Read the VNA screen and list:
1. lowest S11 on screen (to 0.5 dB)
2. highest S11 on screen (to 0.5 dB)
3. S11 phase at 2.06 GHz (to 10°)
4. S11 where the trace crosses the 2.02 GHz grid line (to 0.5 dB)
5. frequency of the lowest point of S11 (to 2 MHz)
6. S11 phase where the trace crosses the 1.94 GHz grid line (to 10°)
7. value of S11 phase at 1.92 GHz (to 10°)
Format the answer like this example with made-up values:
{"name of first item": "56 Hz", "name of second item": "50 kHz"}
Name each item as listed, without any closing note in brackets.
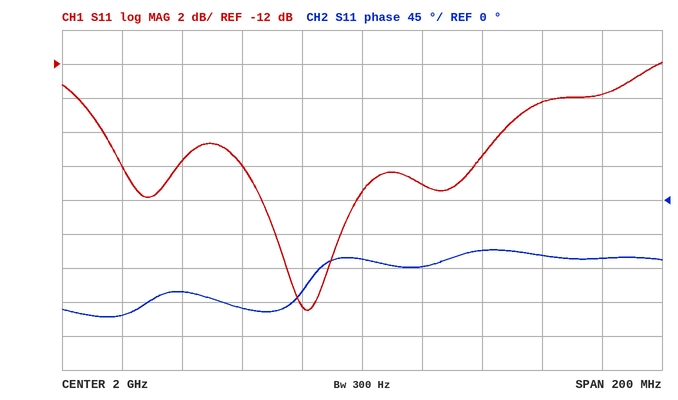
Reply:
{"lowest S11 on screen": "-26.5 dB", "highest S11 on screen": "-12.0 dB", "S11 phase at 2.06 GHz": "-70°", "S11 where the trace crosses the 2.02 GHz grid line": "-19.0 dB", "frequency of the lowest point of S11": "1.982 GHz", "S11 phase where the trace crosses the 1.94 GHz grid line": "-120°", "value of S11 phase at 1.92 GHz": "-150°"}
